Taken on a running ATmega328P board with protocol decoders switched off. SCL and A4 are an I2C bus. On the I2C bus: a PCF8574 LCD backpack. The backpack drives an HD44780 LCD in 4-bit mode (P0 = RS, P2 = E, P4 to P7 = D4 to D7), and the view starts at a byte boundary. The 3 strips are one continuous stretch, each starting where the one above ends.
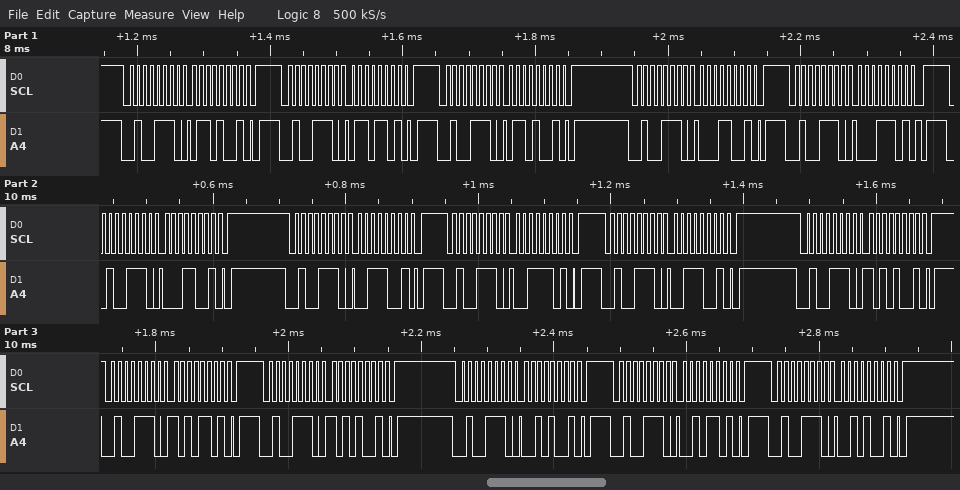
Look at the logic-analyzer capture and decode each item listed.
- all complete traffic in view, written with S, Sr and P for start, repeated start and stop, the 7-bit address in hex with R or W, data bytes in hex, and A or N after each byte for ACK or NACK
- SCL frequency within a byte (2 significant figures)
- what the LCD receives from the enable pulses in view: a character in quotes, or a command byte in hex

S 27W A 69 A P S 27W A 6D A P S 27W A 69 A P S 27W A 19 A P S 27W A 1D A P S 27W A 19 A P S 27W A 39 A P S 27W A 3D A P S 27W A 39 A P S 27W A A9 A P S 27W A AD A P S 27W A A9 A P S 27W A 29 A P S 27W A 2D A P S 27W A 29 A P
100 kHz
'a' ':'
